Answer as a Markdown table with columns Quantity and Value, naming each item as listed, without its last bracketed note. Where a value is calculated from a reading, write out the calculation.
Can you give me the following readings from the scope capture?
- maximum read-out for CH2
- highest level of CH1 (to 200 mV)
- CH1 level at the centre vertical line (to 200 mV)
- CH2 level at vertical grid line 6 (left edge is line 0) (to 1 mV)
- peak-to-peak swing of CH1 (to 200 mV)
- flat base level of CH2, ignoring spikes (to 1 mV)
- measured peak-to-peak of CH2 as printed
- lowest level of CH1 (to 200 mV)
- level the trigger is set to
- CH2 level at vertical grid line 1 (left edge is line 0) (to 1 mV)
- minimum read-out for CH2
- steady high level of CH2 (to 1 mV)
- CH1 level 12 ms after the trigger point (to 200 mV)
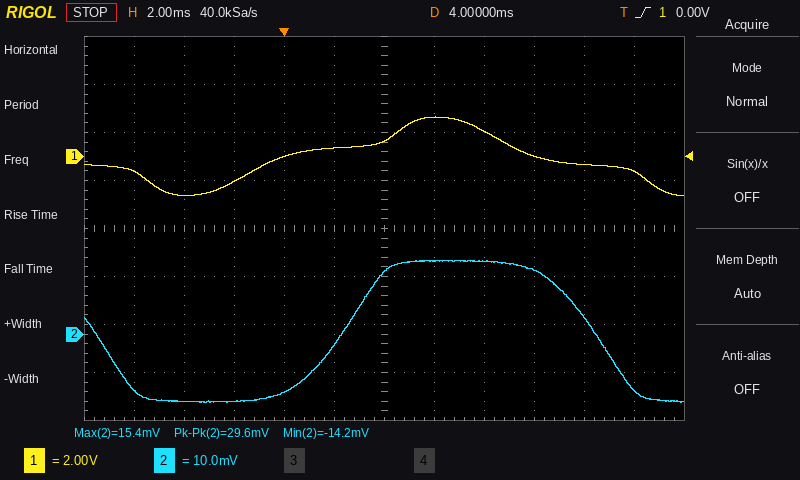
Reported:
| Quantity | Value |
|---|---|
| maximum read-out for CH2 | 15.4 mV |
| highest level of CH1 | 1.6 V |
| CH1 level at the centre vertical line | 600 mV |
| CH2 level at vertical grid line 6 (left edge is line 0) | 13 mV |
| peak-to-peak swing of CH1 | 1.6 V − (-1.6 V) = 3.2 V |
| flat base level of CH2, ignoring spikes | -14 mV |
| measured peak-to-peak of CH2 as printed | 29.6 mV |
| lowest level of CH1 | -1.6 V |
| level the trigger is set to | 0.00 V |
| CH2 level at vertical grid line 1 (left edge is line 0) | -12 mV |
| minimum read-out for CH2 | -14.2 mV |
| steady high level of CH2 | 15 mV |
| CH1 level 12 ms after the trigger point | -400 mV |
